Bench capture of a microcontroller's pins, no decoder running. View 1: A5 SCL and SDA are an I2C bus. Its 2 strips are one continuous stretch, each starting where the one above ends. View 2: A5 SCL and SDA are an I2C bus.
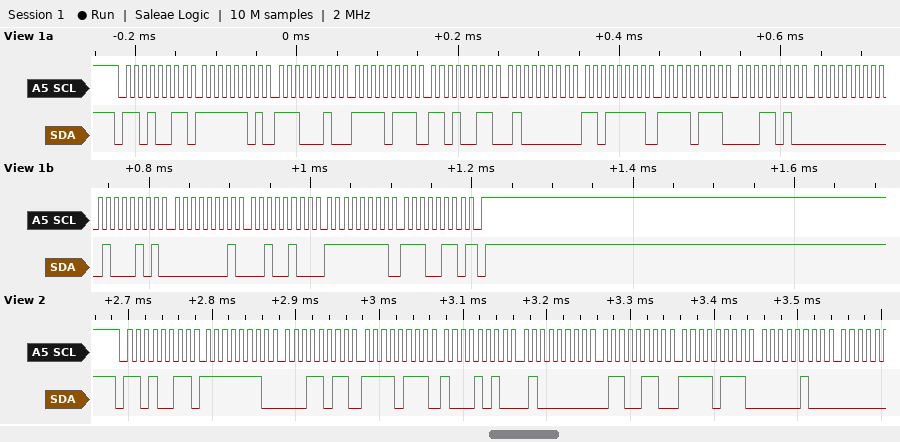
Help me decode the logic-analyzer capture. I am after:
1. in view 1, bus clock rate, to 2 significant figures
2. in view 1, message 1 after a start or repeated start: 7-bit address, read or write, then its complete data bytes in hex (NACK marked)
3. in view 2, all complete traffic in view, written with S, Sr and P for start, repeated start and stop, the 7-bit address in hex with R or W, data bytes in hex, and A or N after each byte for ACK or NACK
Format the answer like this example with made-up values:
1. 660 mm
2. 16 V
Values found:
1. 100 kHz
2. 0x69 read: FD E2 F7 D3 40 DF F7 1A 00 45 01 24 FF E6 NACK
3. S 69R A FE A 1B A F7 A 8A A 40 A 66 A F7 A 04 A
